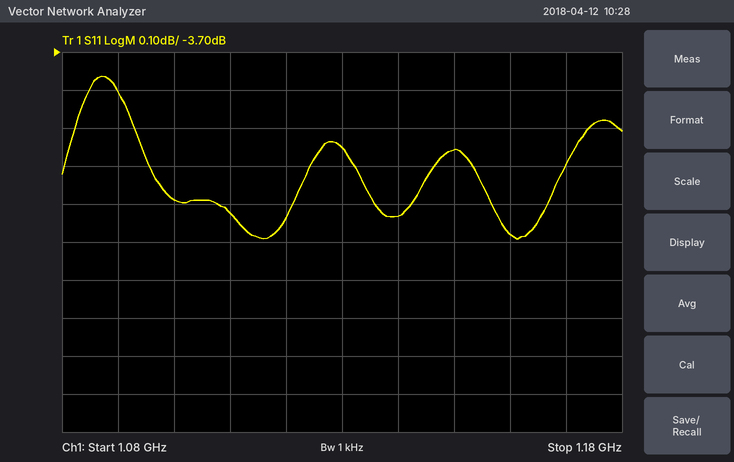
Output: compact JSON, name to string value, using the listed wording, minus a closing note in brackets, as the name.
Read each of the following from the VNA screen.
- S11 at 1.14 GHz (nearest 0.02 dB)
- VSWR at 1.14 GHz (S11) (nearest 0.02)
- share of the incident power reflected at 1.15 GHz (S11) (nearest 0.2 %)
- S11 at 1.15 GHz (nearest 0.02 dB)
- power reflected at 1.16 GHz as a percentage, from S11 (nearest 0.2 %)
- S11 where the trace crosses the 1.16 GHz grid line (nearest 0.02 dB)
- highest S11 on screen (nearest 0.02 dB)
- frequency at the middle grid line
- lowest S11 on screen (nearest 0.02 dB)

{"S11 at 1.14 GHz": "-4.14 dB", "VSWR at 1.14 GHz (S11)": "4.28", "share of the incident power reflected at 1.15 GHz (S11)": "40.2 %", "S11 at 1.15 GHz": "-3.96 dB", "power reflected at 1.16 GHz as a percentage, from S11": "38.2 %", "S11 where the trace crosses the 1.16 GHz grid line": "-4.18 dB", "highest S11 on screen": "-3.76 dB", "frequency at the middle grid line": "1.13 GHz", "lowest S11 on screen": "-4.20 dB"}
